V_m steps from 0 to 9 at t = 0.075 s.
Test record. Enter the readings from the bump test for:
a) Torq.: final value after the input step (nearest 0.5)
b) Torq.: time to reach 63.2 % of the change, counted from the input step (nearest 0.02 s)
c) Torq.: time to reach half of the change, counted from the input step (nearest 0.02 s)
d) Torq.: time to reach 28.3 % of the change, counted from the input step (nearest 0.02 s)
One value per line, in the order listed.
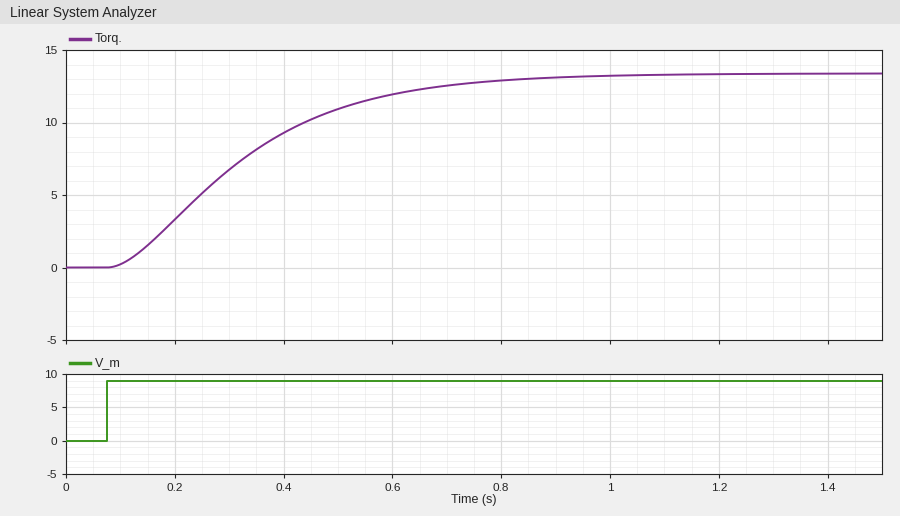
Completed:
13.5
0.28 s
0.22 s
0.14 s
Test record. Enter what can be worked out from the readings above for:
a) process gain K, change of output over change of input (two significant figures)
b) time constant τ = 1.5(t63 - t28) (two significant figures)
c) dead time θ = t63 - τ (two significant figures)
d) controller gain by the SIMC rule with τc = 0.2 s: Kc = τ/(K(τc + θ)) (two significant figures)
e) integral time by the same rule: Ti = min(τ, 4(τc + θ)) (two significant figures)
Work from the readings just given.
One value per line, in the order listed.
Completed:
1.5
0.21 s
0.070 s
0.52
0.21 s
